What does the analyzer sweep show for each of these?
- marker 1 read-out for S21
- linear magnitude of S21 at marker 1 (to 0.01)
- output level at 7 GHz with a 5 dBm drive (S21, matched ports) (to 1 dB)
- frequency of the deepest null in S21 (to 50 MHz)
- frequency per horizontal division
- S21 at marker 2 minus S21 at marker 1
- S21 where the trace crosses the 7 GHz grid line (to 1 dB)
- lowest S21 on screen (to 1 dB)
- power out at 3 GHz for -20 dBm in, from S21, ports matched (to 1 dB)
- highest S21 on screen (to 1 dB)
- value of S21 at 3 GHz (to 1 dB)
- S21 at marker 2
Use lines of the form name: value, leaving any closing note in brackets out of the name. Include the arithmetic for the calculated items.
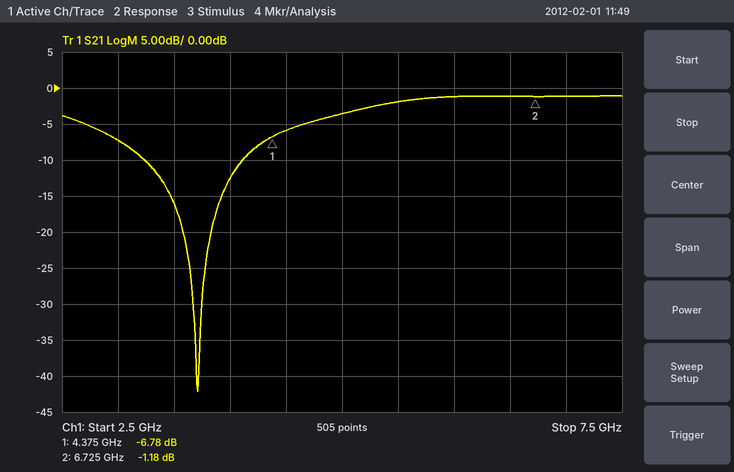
marker 1 read-out for S21: -6.78 dB
linear magnitude of S21 at marker 1: 10^(-6.78/20) ≈ 0.46
output level at 7 GHz with a 5 dBm drive (S21, matched ports): 5 dBm + (-1 dB) = 4 dBm
frequency of the deepest null in S21: 3.70 GHz
frequency per horizontal division: 500 MHz
S21 at marker 2 minus S21 at marker 1: -1.18 − (-6.78) = 5.60 dB
S21 where the trace crosses the 7 GHz grid line: -1 dB
lowest S21 on screen: -42 dB
power out at 3 GHz for -20 dBm in, from S21, ports matched: -20 dBm + (-7 dB) = -27 dBm
highest S21 on screen: -1 dB
value of S21 at 3 GHz: -7 dB
S21 at marker 2: -1.18 dB
